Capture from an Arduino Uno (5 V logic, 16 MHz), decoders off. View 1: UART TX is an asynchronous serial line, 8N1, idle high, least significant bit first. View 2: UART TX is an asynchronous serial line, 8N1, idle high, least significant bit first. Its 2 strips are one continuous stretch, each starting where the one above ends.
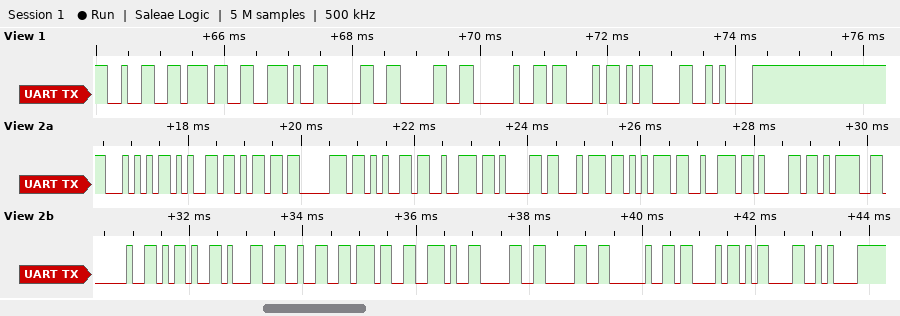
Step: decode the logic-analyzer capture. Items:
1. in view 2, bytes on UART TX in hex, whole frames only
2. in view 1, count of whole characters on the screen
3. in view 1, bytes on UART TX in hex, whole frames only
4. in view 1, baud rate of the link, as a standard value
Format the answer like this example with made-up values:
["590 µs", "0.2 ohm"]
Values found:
["54 65 6D 70 65 72 61 74 75 72 61 3D 20 2D 31 32 37 2E 30 30 20 43 0D 0A", "9", "32 37 2E 30 30 20 43 0D 0A", "9600 baud"]
